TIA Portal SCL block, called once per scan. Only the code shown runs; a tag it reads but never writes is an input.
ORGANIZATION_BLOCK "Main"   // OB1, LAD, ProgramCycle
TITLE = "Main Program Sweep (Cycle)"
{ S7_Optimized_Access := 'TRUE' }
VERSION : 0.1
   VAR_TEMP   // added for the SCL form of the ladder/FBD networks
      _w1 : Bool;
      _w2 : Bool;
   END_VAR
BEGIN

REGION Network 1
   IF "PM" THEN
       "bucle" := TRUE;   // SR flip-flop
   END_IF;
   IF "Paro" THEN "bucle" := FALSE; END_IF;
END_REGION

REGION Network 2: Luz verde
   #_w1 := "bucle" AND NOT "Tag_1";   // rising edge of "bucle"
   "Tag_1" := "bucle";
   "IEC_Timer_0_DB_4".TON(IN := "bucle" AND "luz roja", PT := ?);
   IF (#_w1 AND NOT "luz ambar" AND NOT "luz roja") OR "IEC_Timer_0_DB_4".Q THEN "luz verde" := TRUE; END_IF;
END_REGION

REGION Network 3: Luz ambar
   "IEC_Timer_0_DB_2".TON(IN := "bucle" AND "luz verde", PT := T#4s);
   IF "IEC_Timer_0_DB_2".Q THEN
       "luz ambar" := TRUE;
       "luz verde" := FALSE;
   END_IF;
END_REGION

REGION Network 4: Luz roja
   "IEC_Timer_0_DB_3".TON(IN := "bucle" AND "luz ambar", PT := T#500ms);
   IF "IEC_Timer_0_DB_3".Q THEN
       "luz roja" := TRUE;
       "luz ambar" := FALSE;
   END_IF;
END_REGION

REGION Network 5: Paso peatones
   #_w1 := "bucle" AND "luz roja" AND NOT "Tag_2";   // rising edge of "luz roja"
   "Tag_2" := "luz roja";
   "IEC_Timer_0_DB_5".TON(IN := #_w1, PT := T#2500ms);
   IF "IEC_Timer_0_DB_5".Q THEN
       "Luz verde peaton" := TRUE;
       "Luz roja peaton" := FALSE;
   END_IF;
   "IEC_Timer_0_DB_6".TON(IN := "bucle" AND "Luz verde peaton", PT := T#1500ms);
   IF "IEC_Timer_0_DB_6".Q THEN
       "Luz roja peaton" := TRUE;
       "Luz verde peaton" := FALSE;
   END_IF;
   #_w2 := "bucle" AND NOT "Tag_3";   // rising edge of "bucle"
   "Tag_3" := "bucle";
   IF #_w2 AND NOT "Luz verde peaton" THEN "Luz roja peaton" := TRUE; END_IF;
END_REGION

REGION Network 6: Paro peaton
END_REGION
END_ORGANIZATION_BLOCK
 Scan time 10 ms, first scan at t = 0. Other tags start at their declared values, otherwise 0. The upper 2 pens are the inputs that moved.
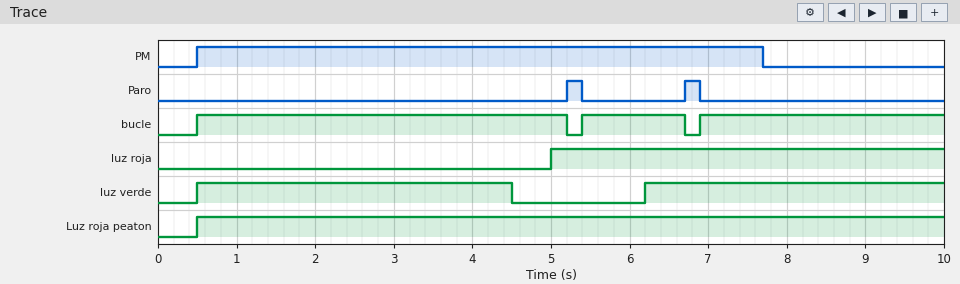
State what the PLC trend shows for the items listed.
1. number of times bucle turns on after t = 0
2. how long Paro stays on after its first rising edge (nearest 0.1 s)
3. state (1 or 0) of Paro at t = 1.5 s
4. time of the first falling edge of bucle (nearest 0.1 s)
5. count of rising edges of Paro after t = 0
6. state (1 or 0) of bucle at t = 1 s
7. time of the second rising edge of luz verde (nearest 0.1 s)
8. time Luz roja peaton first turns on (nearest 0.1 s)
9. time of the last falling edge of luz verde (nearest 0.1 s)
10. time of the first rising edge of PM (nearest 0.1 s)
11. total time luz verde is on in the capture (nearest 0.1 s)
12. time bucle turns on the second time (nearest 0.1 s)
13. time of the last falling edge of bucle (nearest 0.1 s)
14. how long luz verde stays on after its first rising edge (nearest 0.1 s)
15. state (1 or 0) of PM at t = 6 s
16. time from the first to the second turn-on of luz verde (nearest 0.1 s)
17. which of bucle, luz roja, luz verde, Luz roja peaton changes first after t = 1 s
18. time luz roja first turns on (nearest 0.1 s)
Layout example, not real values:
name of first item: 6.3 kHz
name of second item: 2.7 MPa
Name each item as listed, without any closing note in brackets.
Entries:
number of times bucle turns on after t = 0: 3
how long Paro stays on after its first rising edge: 0.2 s
state (1 or 0) of Paro at t = 1.5 s: 0
time of the first falling edge of bucle: 5.2 s
count of rising edges of Paro after t = 0: 2
state (1 or 0) of bucle at t = 1 s: 1
time of the second rising edge of luz verde: 6.2 s
time Luz roja peaton first turns on: 0.5 s
time of the last falling edge of luz verde: 4.5 s
time of the first rising edge of PM: 0.5 s
total time luz verde is on in the capture: 7.8 s
time bucle turns on the second time: 5.4 s
time of the last falling edge of bucle: 6.7 s
how long luz verde stays on after its first rising edge: 4.0 s
state (1 or 0) of PM at t = 6 s: 1
time from the first to the second turn-on of luz verde: 5.7 s
which of bucle, luz roja, luz verde, Luz roja peaton changes first after t = 1 s: luz verde
time luz roja first turns on: 5.0 s
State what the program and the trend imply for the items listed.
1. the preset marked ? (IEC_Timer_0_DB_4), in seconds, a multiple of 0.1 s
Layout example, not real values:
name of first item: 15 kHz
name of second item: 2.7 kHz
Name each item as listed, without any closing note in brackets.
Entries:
the preset marked ? (IEC_Timer_0_DB_4), in seconds, a multiple of 0.1 s: 0.8 s
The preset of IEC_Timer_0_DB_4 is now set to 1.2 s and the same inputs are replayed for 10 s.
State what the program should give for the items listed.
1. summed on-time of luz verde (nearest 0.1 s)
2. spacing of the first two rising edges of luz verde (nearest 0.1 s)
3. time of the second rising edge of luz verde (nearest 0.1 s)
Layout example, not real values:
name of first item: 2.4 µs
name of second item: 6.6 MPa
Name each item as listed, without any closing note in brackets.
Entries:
summed on-time of luz verde: 7.4 s
spacing of the first two rising edges of luz verde: 6.1 s
time of the second rising edge of luz verde: 6.6 s
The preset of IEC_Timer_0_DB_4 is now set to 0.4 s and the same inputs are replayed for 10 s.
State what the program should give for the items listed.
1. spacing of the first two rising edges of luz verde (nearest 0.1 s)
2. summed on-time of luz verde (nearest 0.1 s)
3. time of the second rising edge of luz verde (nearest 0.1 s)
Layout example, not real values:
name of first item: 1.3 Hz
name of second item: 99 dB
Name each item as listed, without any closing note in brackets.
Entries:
spacing of the first two rising edges of luz verde: 5.3 s
summed on-time of luz verde: 8.2 s
time of the second rising edge of luz verde: 5.8 s
